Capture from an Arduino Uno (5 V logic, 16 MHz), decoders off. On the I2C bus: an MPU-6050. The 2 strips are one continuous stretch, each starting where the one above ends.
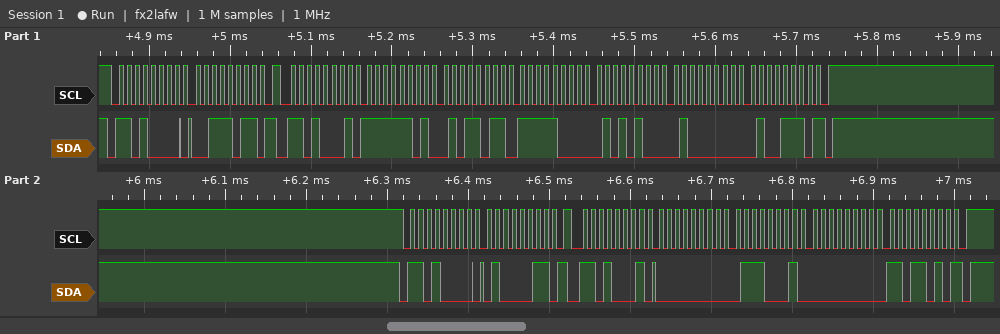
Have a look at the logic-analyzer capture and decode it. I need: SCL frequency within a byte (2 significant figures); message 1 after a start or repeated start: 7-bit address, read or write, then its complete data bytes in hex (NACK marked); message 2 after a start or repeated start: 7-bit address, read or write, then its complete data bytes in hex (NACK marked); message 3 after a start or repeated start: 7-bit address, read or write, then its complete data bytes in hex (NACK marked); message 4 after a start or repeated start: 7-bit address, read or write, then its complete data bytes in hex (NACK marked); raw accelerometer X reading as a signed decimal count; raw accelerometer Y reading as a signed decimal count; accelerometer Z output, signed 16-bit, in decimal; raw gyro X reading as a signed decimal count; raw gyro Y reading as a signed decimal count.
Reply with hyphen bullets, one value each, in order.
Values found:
- 100 kHz
- 0x68 write: 3B
- 0x68 read: FD 5B F8 54 40 4E NACK
- 0x68 write: 43
- 0x68 read: 00 71 00 DA NACK
- -677
- -1964
- 16462
- 113
- 218
